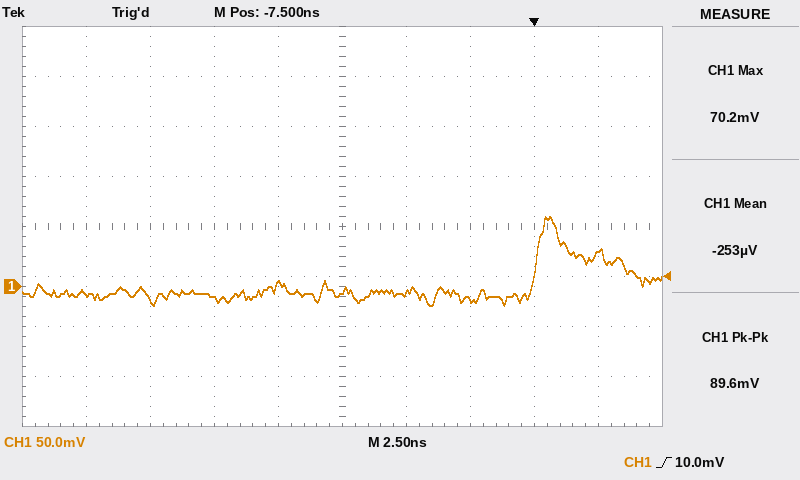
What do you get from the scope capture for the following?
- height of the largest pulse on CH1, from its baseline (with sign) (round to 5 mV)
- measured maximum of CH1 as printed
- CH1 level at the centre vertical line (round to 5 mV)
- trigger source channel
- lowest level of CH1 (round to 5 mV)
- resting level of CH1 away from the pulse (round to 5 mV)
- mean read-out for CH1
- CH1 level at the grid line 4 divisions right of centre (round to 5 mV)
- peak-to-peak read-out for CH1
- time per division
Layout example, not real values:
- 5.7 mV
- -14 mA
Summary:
- +75 mV
- 70.2 mV
- -5 mV
- CH1
- -20 mV
- -5 mV
- -253 µV
- 35 mV
- 89.6 mV
- 2.5 ns
